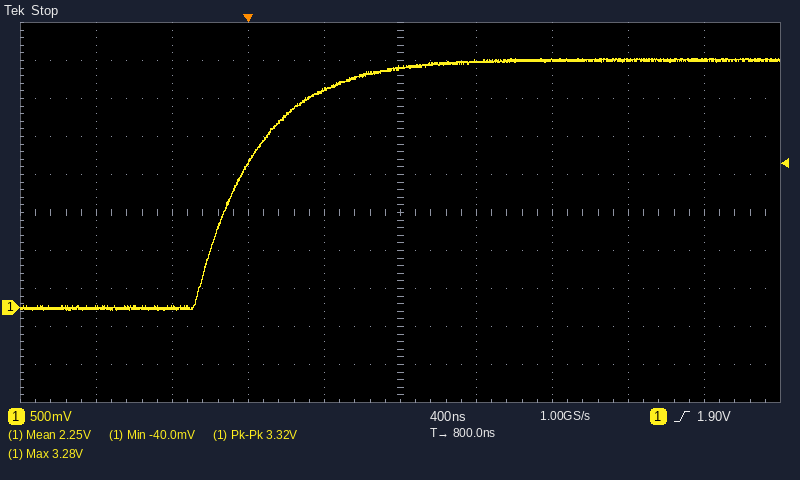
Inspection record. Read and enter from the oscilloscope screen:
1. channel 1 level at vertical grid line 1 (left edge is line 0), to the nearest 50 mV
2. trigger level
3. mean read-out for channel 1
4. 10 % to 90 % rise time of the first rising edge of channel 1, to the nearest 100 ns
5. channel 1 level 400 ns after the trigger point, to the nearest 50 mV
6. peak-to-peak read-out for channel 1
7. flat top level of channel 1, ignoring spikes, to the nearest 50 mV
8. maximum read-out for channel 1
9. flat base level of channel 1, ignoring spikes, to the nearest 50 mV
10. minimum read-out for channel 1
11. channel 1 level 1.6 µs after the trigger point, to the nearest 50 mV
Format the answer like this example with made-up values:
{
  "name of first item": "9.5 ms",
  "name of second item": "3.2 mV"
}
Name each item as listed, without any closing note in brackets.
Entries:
{
  "channel 1 level at vertical grid line 1 (left edge is line 0), to the nearest 50 mV": "0 mV",
  "trigger level": "1.90 V",
  "mean read-out for channel 1": "2.25 V",
  "10 % to 90 % rise time of the first rising edge of channel 1, to the nearest 100 ns": "700 ns",
  "channel 1 level 400 ns after the trigger point, to the nearest 50 mV": "2.85 V",
  "peak-to-peak read-out for channel 1": "3.32 V",
  "flat top level of channel 1, ignoring spikes, to the nearest 50 mV": "3.25 V",
  "maximum read-out for channel 1": "3.28 V",
  "flat base level of channel 1, ignoring spikes, to the nearest 50 mV": "0 mV",
  "minimum read-out for channel 1": "-40.0 mV",
  "channel 1 level 1.6 µs after the trigger point, to the nearest 50 mV": "3.25 V"
}
